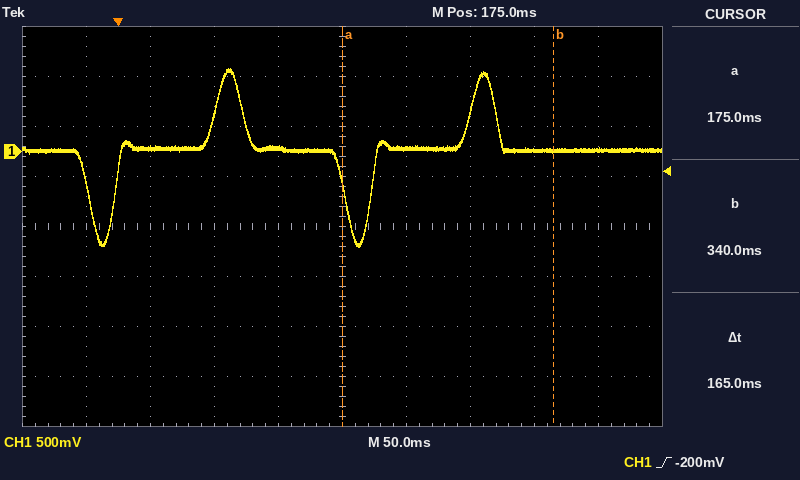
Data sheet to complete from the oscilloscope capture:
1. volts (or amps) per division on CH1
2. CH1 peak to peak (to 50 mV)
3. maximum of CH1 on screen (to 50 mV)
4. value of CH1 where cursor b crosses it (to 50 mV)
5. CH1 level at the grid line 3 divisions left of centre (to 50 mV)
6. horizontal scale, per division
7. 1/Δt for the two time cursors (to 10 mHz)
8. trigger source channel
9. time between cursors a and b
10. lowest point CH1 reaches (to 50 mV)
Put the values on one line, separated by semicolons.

500 mV; 1.80 V; 850 mV; 0 mV; 50 mV; 50 ms; 6.06 Hz; CH1; 165 ms; -950 mV
